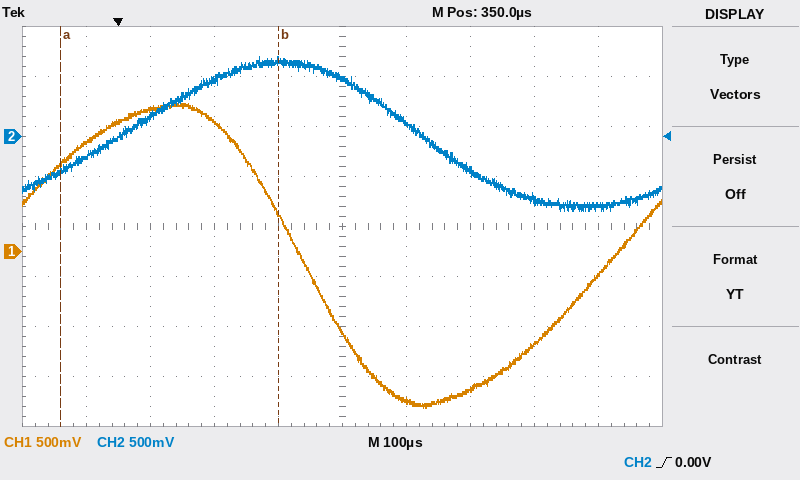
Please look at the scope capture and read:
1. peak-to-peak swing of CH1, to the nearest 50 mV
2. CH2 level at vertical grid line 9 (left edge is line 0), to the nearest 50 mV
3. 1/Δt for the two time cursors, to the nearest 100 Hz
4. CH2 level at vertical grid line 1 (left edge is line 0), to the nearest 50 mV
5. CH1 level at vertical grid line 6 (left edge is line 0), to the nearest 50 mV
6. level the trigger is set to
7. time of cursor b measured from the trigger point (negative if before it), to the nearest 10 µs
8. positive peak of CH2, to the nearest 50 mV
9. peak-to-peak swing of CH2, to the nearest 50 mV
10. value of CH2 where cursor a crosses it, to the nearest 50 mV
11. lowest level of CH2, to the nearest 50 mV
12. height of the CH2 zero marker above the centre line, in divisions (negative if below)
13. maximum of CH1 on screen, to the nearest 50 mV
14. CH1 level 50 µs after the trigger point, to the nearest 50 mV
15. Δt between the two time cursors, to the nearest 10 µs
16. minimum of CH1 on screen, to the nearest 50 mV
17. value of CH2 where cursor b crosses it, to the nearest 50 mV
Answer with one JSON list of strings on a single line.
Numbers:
["3.05 V", "-700 mV", "2.9 kHz", "-200 mV", "-1.50 V", "0.00 V", "+250 µs", "800 mV", "1.55 V", "-350 mV", "-750 mV", "+1.8 div", "1.50 V", "1.40 V", "340 µs", "-1.55 V", "750 mV"]
